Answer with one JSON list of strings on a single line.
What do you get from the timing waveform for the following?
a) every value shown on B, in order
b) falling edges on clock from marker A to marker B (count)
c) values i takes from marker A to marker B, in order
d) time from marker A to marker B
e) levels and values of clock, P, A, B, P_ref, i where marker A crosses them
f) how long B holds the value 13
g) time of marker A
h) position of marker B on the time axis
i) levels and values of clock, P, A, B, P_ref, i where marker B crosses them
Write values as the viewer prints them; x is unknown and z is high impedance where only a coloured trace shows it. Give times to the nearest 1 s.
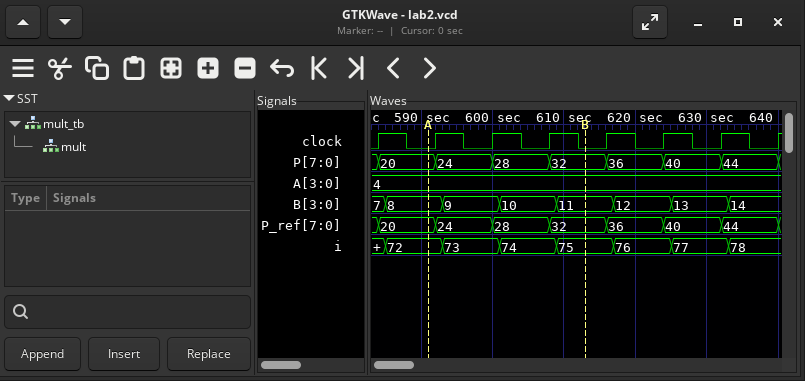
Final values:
["7, 8, 9, 10, 11, 12, 13, 14", "3", "72, 73, 74, 75", "22 s", "clock=0, P=20, A=4, B=8, P_ref=20, i=72", "8 s", "591 s", "613 s", "clock=0, P=32, A=4, B=11, P_ref=32, i=75"]
